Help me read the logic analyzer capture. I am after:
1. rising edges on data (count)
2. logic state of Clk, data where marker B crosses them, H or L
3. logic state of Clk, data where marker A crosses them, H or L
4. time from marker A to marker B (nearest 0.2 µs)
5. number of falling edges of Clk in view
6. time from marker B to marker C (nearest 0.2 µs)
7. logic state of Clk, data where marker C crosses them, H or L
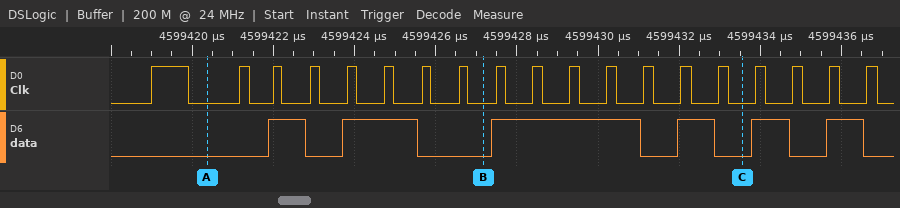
6
Clk=L, data=L
Clk=L, data=L
6.8 µs
19
6.4 µs
Clk=L, data=L
